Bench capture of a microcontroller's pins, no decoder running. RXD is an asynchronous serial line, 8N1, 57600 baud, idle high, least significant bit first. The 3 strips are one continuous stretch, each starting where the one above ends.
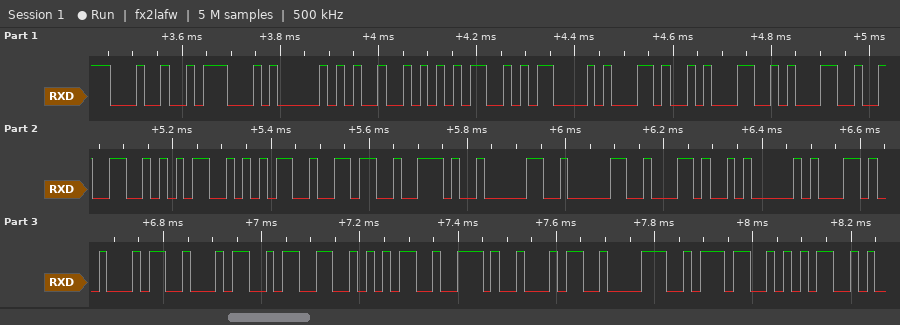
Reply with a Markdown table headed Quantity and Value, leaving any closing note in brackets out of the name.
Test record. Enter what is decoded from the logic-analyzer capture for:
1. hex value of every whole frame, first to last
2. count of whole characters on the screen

| Quantity | Value |
|---|---|
| hex value of every whole frame, first to last | 24 47 50 52 4D 43 2C 31 31 32 35 35 36 2E 30 30 2C 41 2C 34 34 33 35 2E 34 38 37 35 |
| count of whole characters on the screen | 28 |
